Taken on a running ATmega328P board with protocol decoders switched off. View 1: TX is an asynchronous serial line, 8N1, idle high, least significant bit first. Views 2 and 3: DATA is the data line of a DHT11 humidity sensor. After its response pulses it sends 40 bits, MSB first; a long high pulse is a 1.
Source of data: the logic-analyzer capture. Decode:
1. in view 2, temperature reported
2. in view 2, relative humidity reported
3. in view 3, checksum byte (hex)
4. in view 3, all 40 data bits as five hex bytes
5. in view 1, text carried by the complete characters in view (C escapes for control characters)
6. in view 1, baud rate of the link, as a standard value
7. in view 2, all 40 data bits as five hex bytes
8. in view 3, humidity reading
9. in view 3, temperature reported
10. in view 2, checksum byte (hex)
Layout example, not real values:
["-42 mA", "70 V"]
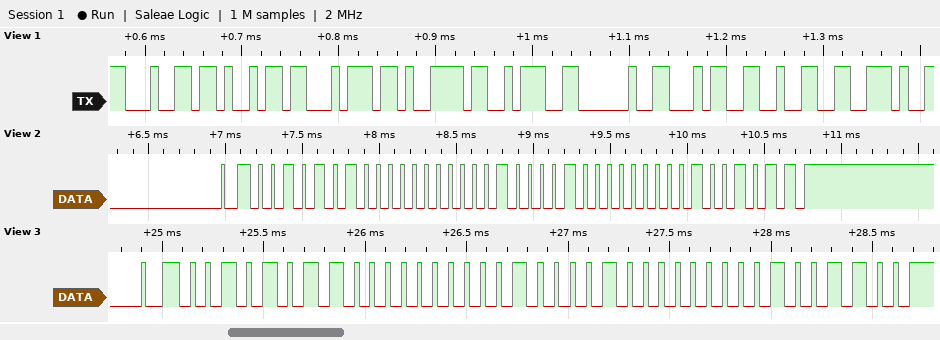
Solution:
["33.0 °C", "42 %", "0x4C", "2B 00 21 00 4C", "\"dity: 42.\"", "115200 baud", "2A 00 21 00 4B", "43 %", "33.0 °C", "0x4B"]
